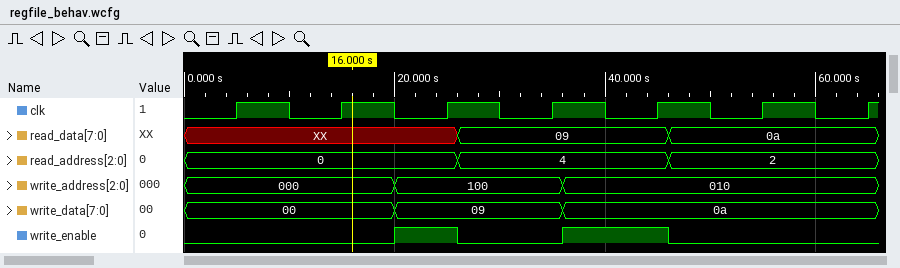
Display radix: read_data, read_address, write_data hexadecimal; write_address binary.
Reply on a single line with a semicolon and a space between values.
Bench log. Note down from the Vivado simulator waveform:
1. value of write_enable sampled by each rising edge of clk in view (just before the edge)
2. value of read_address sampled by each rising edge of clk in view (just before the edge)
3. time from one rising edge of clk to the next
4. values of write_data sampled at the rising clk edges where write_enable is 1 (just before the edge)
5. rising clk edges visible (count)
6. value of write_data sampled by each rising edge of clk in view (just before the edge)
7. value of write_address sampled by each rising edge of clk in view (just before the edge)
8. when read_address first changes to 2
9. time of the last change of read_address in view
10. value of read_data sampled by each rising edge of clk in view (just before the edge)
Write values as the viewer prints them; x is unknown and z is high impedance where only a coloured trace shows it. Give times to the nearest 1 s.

0 0 1 0 1 0 0; 0, 0, 0, 4, 4, 2, 2; 10 s; 09, 0a; 7; 00, 00, 09, 09, 0a, 0a, 0a; 000, 000, 100, 100, 010, 010, 010; 46 s; 46 s; XX, XX, XX, 09, 09, 0a, 0a
